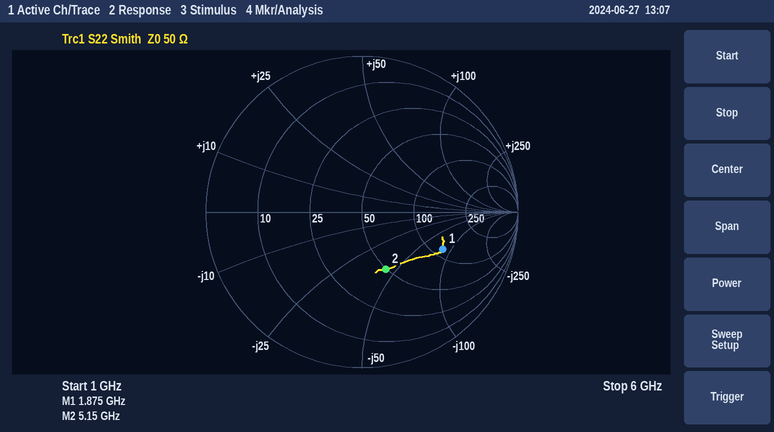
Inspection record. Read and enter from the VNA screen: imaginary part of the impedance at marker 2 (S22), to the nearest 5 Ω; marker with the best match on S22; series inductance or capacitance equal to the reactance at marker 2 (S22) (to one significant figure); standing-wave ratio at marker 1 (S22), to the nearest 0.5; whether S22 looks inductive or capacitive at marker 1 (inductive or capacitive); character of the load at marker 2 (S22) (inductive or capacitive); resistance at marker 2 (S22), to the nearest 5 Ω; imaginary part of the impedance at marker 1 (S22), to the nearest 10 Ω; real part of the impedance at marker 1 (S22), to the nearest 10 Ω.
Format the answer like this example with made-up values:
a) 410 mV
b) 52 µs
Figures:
a) -45 Ω
b) marker 2
c) 700 fF
d) 3.5
e) capacitive
f) capacitive
g) 50 Ω
h) -80 Ω
i) 120 Ω
